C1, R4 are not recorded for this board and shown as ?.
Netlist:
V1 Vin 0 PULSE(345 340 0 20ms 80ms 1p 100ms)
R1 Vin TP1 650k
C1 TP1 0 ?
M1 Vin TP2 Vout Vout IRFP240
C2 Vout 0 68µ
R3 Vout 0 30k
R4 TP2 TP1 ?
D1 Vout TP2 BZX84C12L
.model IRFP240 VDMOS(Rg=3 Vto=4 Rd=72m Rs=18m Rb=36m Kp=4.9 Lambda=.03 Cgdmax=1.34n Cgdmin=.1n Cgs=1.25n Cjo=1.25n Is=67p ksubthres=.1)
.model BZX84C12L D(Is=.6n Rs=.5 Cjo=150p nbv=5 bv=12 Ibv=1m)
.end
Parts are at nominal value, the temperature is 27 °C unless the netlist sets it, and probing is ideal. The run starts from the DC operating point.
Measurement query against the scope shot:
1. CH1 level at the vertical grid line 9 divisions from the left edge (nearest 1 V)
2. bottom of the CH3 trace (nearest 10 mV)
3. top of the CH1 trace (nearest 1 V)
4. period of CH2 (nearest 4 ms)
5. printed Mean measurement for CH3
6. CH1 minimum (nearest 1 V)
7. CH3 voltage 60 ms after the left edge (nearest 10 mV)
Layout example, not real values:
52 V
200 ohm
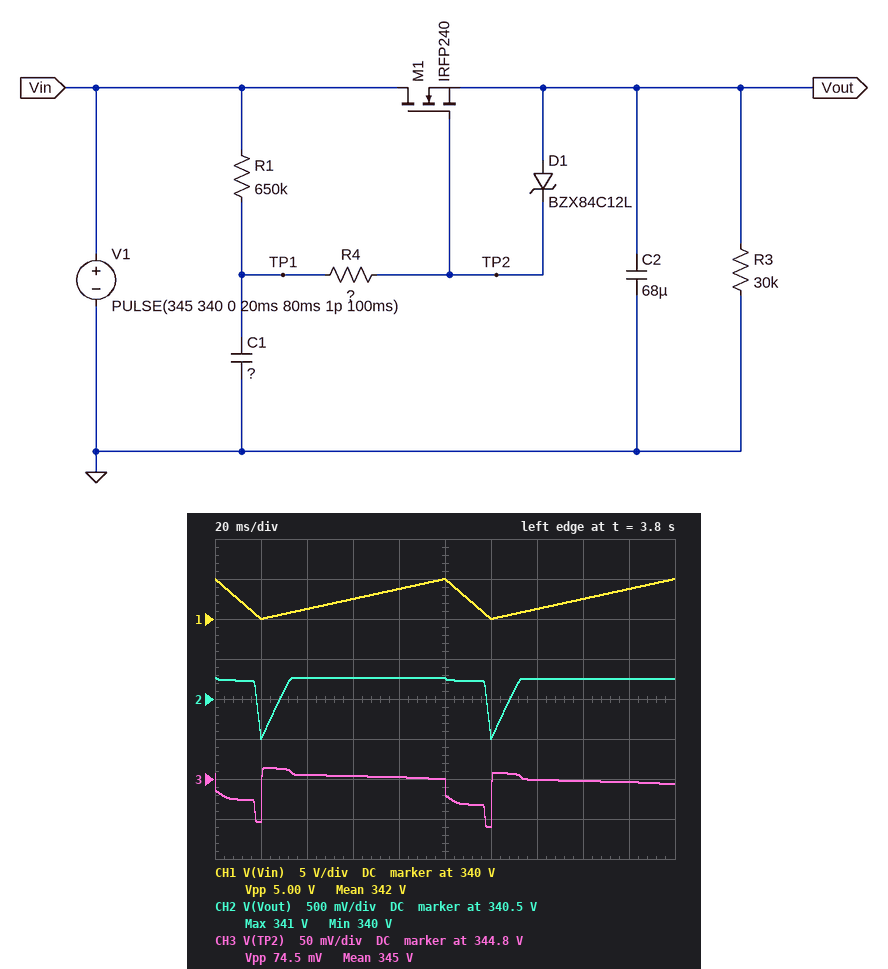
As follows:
344 V
344.69 V
345 V
100 ms
345 V
340 V
344.75 V
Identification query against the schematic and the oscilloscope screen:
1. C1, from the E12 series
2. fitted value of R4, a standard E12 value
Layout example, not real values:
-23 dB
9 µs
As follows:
56 µF
82 kΩ
